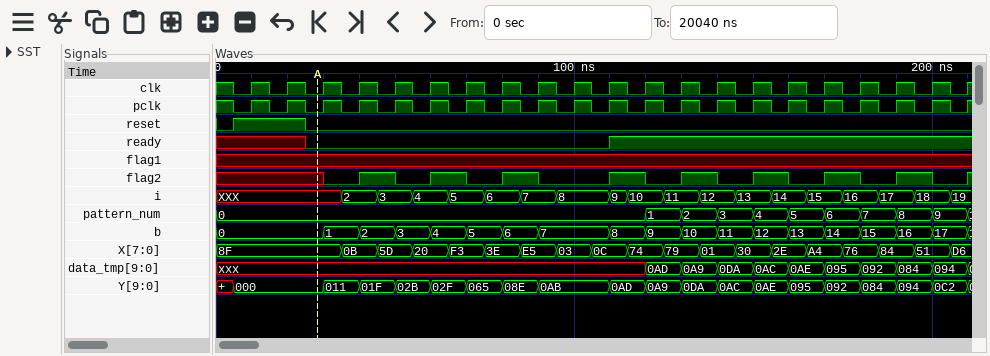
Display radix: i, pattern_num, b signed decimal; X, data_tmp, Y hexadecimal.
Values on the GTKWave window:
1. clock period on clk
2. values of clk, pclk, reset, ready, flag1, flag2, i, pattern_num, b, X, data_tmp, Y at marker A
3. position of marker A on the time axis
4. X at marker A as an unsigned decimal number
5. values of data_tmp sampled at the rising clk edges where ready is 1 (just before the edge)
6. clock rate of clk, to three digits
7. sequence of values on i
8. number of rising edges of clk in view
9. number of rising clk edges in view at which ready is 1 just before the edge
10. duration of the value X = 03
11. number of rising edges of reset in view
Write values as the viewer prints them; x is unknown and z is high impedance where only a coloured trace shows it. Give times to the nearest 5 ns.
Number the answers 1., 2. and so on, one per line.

1. 10 ns
2. clk=0, pclk=0, reset=0, ready=0, flag1=x, flag2=x, i=XXX, pattern_num=0, b=0, X=8F, data_tmp=xxx, Y=000
3. 30 ns
4. 143
5. xxx, 0AD, 0A9, 0DA, 0AC, 0AE, 095, 092, 084, 094
6. 100 MHz
7. XXX, 2, 3, 4, 5, 6, 7, 8, 9, 10, 11, 12, 13, 14, 15, 16, 17, 18, 19
8. 21
9. 10
10. 10 ns
11. 1
